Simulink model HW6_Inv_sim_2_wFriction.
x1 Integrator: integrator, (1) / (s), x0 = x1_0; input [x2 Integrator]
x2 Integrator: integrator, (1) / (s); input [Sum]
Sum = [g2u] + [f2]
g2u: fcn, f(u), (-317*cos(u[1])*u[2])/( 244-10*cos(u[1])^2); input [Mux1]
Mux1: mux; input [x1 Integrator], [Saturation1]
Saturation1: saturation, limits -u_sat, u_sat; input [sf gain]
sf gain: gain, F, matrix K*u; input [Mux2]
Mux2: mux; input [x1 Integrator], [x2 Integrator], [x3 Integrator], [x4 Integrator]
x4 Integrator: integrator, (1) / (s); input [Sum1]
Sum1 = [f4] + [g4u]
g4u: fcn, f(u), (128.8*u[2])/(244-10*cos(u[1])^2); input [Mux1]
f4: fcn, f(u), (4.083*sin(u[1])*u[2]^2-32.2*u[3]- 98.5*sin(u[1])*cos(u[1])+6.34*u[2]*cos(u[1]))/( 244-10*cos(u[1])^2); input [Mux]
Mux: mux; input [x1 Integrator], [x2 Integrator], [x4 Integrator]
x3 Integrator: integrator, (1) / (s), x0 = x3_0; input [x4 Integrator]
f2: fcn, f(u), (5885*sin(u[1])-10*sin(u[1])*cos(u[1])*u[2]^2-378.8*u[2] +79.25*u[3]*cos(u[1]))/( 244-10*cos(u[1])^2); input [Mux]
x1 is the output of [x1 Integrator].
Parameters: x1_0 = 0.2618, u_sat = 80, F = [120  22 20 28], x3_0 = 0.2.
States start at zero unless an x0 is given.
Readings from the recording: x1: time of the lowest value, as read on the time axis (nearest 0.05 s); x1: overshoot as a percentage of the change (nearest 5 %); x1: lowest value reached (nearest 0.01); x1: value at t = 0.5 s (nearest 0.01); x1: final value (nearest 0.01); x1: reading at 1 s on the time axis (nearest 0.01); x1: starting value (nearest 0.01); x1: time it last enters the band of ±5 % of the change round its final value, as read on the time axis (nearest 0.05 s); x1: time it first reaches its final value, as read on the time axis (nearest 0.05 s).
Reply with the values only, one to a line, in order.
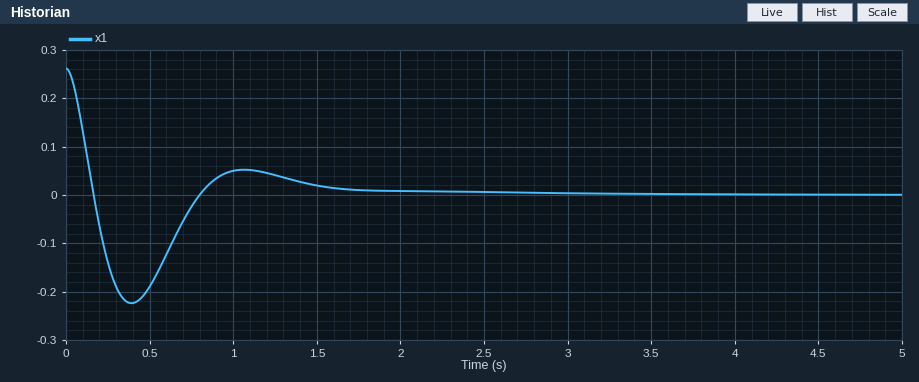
0.40 s
85 %
-0.22
-0.19
0.00
0.05
0.26
1.65 s
0.15 s
